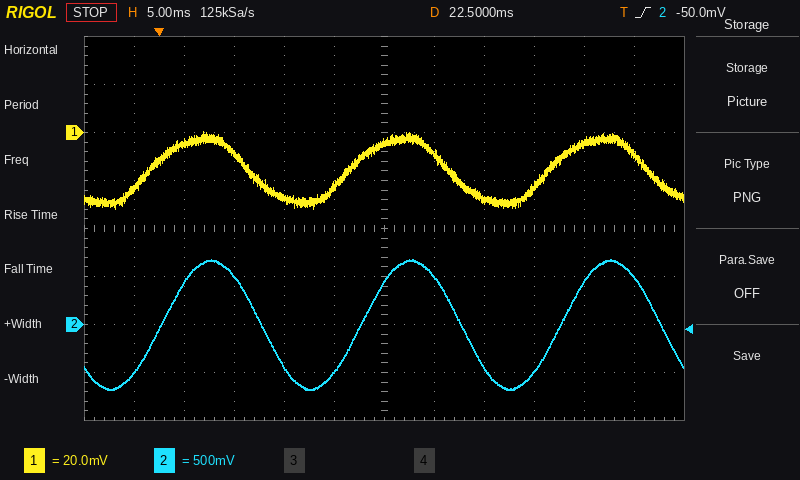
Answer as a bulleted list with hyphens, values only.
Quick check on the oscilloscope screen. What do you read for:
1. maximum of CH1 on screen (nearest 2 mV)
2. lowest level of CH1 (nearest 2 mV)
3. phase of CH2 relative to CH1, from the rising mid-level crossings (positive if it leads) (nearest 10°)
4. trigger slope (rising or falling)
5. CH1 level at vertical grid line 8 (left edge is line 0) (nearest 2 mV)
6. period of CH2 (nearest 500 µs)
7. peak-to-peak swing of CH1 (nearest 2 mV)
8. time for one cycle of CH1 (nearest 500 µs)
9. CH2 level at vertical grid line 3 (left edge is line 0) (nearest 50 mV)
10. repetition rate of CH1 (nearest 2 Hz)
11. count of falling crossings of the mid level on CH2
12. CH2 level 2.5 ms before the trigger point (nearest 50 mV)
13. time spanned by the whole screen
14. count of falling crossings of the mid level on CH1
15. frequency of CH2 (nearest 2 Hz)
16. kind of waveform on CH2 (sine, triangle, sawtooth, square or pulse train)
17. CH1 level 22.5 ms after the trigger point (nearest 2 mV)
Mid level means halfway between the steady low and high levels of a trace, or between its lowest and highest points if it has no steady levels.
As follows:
- 0 mV
- -32 mV
- -20°
- rising
- -28 mV
- 20.0 ms
- 32 mV
- 20.0 ms
- 500 mV
- 50 Hz
- 3
- -500 mV
- 60 ms
- 3
- 50 Hz
- sine
- -4 mV
